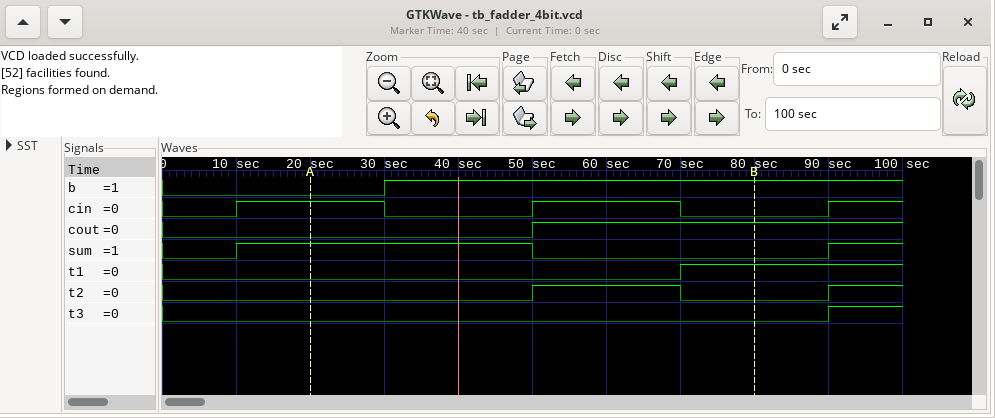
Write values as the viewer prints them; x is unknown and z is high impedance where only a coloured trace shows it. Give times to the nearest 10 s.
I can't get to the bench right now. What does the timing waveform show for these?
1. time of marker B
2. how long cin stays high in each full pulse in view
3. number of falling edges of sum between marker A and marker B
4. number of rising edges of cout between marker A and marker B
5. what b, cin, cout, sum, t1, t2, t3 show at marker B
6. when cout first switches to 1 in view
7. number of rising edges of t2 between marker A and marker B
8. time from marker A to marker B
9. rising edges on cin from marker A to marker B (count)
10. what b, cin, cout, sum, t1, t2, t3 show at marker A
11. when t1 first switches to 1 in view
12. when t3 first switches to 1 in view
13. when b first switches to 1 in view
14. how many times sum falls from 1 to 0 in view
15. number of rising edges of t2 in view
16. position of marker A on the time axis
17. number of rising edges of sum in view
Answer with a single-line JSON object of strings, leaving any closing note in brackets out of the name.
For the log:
{"time of marker B": "80 s", "how long cin stays high in each full pulse in view": "20 s, 20 s", "number of falling edges of sum between marker A and marker B": "1", "number of rising edges of cout between marker A and marker B": "1", "what b, cin, cout, sum, t1, t2, t3 show at marker B": "b=1, cin=0, cout=1, sum=0, t1=1, t2=0, t3=0", "when cout first switches to 1 in view": "50 s", "number of rising edges of t2 between marker A and marker B": "1", "time from marker A to marker B": "60 s", "rising edges on cin from marker A to marker B": "1", "what b, cin, cout, sum, t1, t2, t3 show at marker A": "b=0, cin=1, cout=0, sum=1, t1=0, t2=0, t3=0", "when t1 first switches to 1 in view": "70 s", "when t3 first switches to 1 in view": "90 s", "when b first switches to 1 in view": "30 s", "how many times sum falls from 1 to 0 in view": "1", "number of rising edges of t2 in view": "2", "position of marker A on the time axis": "20 s", "number of rising edges of sum in view": "2"}
